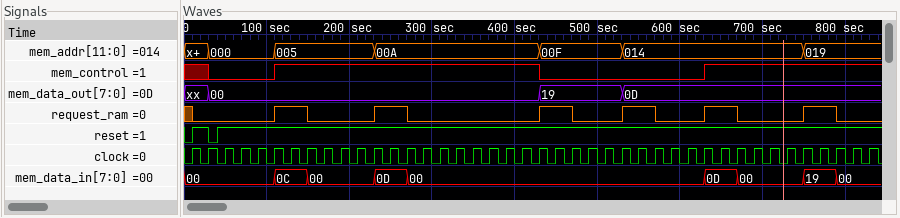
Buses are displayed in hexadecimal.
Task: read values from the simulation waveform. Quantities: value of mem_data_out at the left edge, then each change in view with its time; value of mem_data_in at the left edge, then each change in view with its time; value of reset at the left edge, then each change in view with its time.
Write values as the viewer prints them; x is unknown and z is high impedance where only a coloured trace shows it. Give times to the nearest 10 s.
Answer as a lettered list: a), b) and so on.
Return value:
a) xx, 00 at 30 s, 19 at 430 s, 0D at 530 s
b) 00, 0C at 110 s, 00 at 150 s, 0D at 230 s, 00 at 270 s, 0D at 630 s, 00 at 670 s, 19 at 750 s, 00 at 790 s
c) 0, 1 at 10 s, 0 at 30 s, 1 at 40 s
